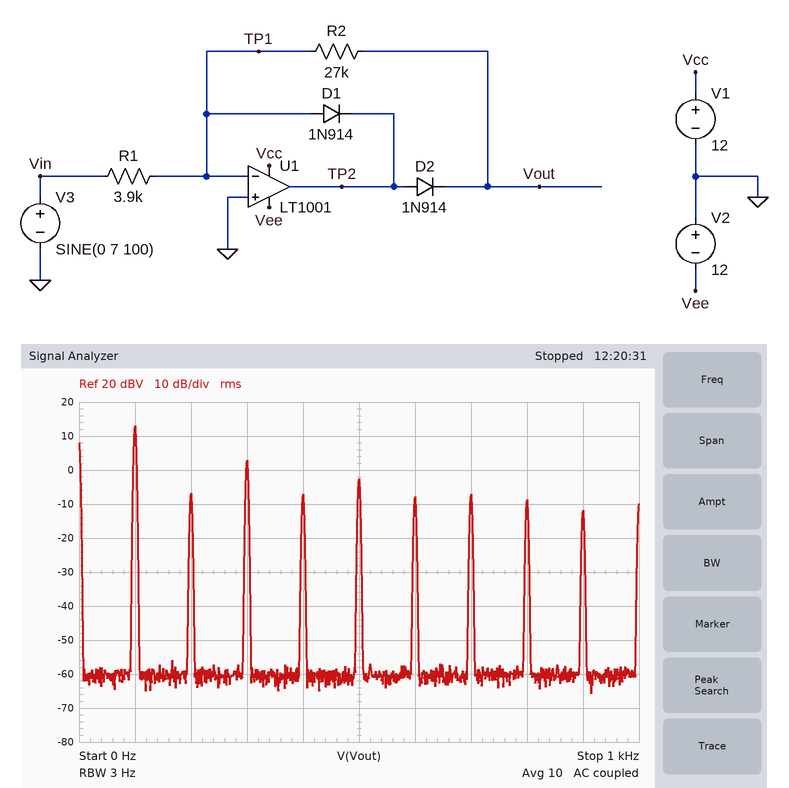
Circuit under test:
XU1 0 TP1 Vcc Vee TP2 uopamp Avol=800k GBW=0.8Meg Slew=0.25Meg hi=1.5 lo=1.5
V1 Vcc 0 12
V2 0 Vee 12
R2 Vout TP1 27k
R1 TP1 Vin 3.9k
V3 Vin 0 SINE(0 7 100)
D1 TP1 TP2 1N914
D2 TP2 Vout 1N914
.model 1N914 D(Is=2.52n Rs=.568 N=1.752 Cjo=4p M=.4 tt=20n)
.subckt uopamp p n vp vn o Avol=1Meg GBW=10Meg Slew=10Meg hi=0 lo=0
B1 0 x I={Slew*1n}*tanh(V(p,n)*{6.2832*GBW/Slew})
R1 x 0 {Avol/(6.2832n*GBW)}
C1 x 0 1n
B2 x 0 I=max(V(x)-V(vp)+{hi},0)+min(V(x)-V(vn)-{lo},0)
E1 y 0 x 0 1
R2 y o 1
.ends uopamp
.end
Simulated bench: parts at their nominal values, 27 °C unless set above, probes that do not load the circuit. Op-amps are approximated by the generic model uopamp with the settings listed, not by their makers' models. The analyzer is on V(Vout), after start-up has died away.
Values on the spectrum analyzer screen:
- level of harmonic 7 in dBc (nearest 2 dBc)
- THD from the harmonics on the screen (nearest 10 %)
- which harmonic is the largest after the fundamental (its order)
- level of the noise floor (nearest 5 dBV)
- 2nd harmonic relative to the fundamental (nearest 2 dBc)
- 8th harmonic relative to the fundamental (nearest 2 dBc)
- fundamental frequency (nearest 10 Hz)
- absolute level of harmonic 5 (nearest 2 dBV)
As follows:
-20 dBc
40 %
3
-60 dBV
-20 dBc
-22 dBc
100 Hz
-2 dBV
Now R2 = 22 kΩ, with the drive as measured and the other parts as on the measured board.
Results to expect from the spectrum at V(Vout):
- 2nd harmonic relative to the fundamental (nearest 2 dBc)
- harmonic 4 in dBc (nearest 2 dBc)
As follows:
-18 dBc
-18 dBc
